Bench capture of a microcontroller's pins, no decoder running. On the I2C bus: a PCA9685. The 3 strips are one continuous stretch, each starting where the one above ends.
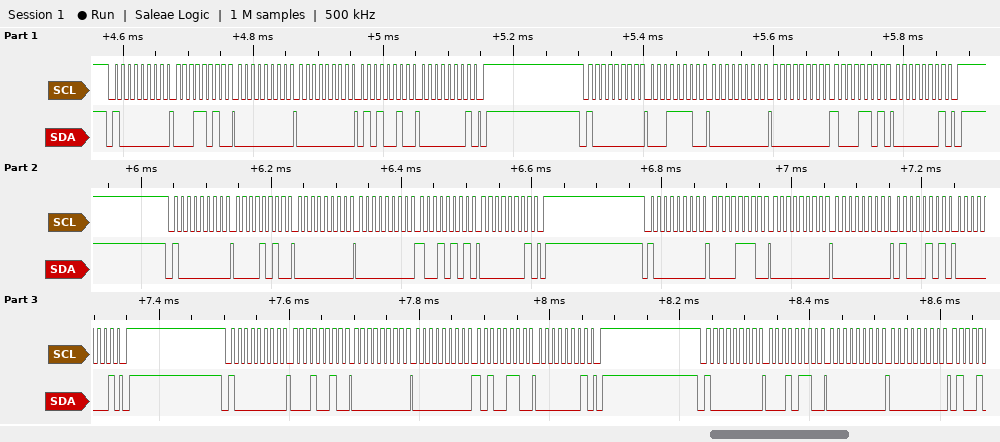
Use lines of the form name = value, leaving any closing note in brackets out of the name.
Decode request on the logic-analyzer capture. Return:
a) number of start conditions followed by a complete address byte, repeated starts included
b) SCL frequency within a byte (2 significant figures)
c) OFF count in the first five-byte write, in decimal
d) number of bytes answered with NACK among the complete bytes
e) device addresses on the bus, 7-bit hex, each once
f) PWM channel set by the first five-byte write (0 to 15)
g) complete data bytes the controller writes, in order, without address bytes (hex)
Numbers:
number of start conditions followed by a complete address byte, repeated starts included = 6
SCL frequency within a byte = 100 kHz
OFF count in the first five-byte write, in decimal = 338
number of bytes answered with NACK among the complete bytes = 0
device addresses on the bus, 7-bit hex, each once = 0x40
PWM channel set by the first five-byte write = 5
complete data bytes the controller writes, in order, without address bytes = 1A 00 00 52 01 1E 00 00 8D 01 0A 00 00 95 01 0E 00 00 45 01 12 00 00 A6 01 16 00 00
